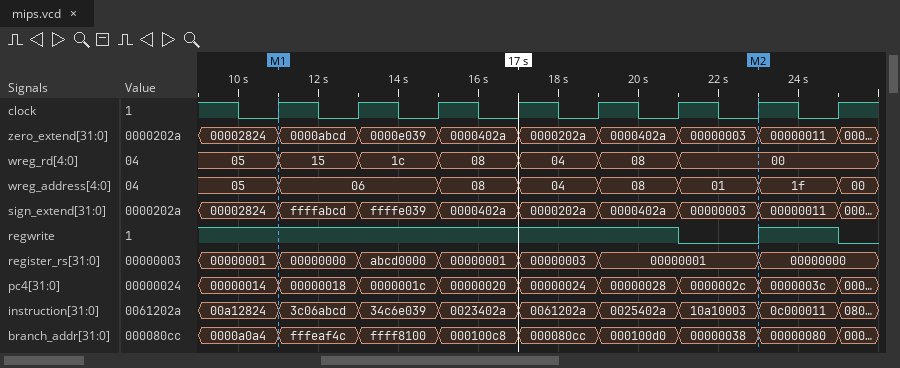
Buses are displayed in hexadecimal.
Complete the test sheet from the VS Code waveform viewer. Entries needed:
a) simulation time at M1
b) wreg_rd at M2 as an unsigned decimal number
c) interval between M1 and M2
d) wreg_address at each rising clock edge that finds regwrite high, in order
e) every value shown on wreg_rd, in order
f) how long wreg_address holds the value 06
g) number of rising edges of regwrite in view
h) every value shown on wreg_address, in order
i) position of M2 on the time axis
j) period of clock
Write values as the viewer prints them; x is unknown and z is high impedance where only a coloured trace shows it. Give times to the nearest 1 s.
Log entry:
11 s
0
12 s
05, 06, 06, 08, 04, 08, 1f
05, 15, 1c, 08, 04, 08, 00
4 s
1
05, 06, 08, 04, 08, 01, 1f, 00
23 s
2 s
